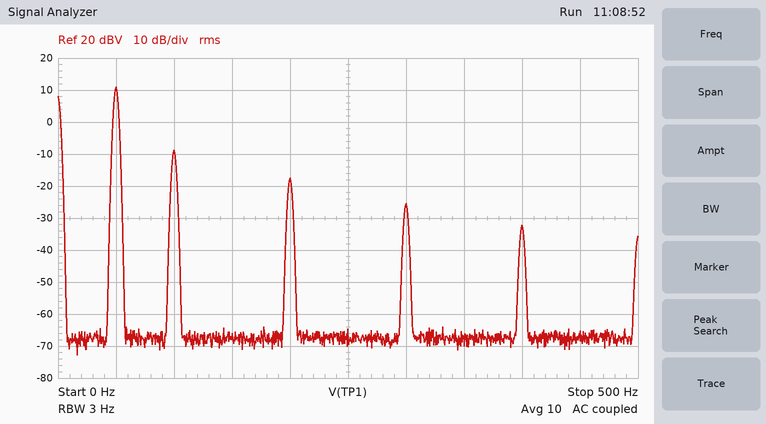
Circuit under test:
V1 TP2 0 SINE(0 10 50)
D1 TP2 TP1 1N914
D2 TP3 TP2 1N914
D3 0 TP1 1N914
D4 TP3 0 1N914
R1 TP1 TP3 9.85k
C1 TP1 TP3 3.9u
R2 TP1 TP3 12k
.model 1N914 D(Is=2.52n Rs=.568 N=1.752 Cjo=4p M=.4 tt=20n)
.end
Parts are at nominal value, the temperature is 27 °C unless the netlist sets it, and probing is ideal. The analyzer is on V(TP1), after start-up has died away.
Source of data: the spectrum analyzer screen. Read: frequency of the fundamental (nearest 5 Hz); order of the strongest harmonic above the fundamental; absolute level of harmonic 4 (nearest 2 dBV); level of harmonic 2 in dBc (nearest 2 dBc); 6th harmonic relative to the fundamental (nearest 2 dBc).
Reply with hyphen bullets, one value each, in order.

- 50 Hz
- 2
- -18 dBV
- -20 dBc
- -36 dBc
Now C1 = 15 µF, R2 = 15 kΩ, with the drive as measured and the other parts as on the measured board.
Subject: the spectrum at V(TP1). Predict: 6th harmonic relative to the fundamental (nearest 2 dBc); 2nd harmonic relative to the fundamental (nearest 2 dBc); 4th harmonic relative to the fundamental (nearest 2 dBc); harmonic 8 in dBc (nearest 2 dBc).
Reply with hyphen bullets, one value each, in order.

- -42 dBc
- -30 dBc
- -38 dBc
- -48 dBc
